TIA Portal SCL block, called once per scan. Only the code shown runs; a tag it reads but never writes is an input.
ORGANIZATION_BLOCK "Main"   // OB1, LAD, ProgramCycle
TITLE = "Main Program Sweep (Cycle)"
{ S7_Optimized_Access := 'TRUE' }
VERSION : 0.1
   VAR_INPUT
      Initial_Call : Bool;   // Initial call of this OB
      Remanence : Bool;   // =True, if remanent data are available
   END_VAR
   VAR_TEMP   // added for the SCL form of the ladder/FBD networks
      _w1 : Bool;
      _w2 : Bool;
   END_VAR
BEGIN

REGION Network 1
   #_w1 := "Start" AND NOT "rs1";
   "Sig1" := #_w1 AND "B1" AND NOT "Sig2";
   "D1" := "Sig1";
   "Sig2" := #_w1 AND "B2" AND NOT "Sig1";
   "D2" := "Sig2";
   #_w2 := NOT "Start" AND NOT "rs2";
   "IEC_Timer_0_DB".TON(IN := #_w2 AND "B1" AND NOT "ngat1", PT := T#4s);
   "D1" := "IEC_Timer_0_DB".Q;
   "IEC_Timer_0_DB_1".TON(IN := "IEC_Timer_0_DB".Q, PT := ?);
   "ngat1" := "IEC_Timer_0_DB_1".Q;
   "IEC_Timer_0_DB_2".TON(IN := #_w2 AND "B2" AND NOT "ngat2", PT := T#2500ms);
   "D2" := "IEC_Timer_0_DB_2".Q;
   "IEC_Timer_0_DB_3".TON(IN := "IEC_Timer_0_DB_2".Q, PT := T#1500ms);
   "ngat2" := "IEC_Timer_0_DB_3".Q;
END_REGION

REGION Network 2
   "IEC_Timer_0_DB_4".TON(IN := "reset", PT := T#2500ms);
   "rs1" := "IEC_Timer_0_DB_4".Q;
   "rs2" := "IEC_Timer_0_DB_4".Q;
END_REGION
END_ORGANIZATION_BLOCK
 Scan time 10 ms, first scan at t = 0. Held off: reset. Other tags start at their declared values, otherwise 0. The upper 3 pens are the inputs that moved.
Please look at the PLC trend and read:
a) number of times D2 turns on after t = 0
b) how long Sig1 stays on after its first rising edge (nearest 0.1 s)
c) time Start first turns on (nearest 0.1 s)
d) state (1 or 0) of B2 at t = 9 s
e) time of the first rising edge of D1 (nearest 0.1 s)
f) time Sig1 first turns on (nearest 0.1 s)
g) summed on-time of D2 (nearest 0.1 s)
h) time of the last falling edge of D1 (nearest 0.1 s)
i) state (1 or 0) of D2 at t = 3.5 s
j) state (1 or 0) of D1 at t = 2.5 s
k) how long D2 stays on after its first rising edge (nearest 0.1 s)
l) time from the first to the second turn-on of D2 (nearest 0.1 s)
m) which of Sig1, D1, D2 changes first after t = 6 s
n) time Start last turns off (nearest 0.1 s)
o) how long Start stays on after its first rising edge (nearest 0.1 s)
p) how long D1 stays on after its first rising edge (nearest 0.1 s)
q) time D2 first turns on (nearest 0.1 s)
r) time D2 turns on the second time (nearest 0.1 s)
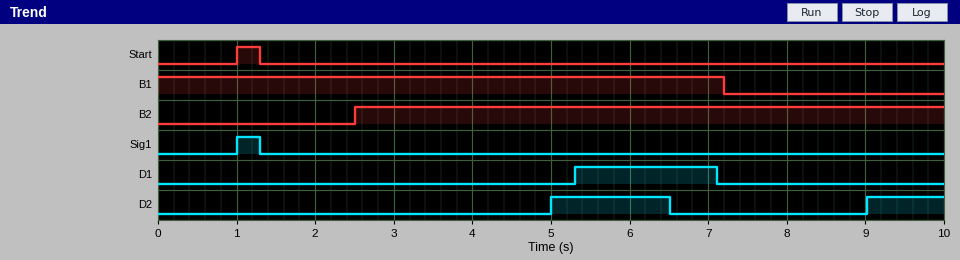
2
0.3 s
1.0 s
1
5.3 s
1.0 s
2.5 s
7.1 s
0
0
1.5 s
4.0 s
D2
1.3 s
0.3 s
1.8 s
5.0 s
9.0 s
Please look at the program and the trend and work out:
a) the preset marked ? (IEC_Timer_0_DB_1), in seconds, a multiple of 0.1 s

1.8 s
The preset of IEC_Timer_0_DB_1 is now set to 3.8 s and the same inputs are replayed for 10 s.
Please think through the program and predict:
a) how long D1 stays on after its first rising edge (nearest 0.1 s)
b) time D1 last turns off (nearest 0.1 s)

1.9 s
7.2 s
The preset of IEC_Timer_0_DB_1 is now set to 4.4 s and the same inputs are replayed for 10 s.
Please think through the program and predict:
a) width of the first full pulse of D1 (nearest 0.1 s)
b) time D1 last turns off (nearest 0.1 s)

1.9 s
7.2 s
